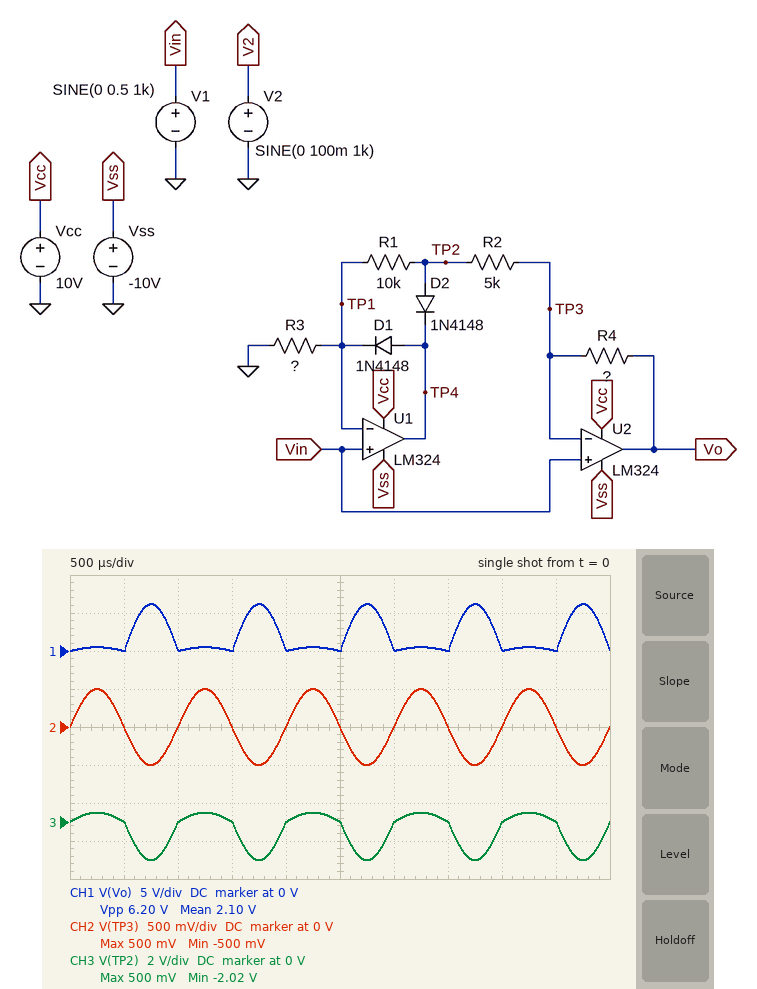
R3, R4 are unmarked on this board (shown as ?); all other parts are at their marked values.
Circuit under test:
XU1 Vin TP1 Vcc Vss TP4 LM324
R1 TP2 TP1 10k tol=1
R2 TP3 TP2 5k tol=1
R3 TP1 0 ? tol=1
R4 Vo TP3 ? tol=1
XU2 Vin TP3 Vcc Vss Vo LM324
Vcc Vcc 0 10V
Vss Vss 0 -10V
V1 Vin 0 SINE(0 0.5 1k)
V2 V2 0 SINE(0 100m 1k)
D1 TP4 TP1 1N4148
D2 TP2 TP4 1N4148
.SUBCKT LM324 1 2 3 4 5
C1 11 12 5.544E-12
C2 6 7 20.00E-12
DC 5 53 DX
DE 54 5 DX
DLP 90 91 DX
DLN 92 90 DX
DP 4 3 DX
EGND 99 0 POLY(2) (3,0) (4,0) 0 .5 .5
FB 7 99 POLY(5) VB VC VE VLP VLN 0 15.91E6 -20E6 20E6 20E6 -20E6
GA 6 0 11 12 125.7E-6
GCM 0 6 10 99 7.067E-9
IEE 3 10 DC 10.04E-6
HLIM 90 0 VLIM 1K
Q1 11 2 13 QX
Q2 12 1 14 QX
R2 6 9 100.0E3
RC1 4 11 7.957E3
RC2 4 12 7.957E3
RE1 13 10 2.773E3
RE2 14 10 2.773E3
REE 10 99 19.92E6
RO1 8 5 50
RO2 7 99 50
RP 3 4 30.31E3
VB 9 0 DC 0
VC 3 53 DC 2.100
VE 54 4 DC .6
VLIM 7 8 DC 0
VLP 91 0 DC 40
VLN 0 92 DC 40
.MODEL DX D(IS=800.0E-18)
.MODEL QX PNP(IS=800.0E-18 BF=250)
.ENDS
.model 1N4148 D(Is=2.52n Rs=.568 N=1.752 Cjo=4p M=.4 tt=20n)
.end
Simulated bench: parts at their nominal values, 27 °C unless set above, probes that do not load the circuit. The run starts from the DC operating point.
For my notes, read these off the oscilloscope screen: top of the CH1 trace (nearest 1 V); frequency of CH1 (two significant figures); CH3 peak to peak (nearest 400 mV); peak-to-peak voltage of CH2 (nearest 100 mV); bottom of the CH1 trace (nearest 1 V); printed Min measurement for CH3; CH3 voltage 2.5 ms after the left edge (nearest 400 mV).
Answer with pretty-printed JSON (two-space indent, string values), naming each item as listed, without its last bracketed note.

{
  "top of the CH1 trace": "6 V",
  "frequency of CH1": "1.0 kHz",
  "CH3 peak to peak": "2.4 V",
  "peak-to-peak voltage of CH2": "1.0 V",
  "bottom of the CH1 trace": "0 V",
  "printed Min measurement for CH3": "-2.02 V",
  "CH3 voltage 2.5 ms after the left edge": "0 V"
}
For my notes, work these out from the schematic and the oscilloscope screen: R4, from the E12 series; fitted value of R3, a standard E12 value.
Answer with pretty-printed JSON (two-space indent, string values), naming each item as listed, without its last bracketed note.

{
  "R4, from the E12 series": "22 kΩ",
  "fitted value of R3, a standard E12 value": "3.3 kΩ"
}
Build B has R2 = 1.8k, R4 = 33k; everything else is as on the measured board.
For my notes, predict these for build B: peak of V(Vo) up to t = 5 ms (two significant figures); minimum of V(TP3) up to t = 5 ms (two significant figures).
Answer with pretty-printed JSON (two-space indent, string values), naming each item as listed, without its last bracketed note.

{
  "peak of V(Vo) up to t = 5 ms": "8.5 V",
  "minimum of V(TP3) up to t = 5 ms": "-1.5 V"
}
